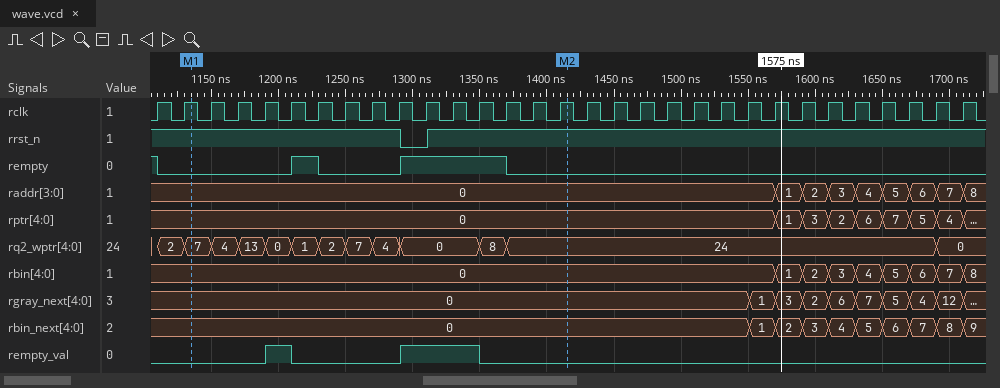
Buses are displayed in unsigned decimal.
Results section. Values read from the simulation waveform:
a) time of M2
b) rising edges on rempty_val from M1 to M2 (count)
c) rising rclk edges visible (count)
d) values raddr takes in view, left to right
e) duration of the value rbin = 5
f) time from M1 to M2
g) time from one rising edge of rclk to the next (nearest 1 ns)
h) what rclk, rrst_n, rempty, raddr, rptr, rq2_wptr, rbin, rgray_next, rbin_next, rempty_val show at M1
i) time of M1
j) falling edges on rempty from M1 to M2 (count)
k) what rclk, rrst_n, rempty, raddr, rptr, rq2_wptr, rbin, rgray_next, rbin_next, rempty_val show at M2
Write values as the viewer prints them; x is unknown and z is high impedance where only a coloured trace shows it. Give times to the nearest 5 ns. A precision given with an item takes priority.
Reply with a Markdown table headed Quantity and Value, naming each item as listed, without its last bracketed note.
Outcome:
| Quantity | Value |
|---|---|
| time of M2 | 1415 ns |
| rising edges on rempty_val from M1 to M2 | 2 |
| rising rclk edges visible | 31 |
| values raddr takes in view, left to right | 0, 1, 2, 3, 4, 5, 6, 7, 8 |
| duration of the value rbin = 5 | 20 ns |
| time from M1 to M2 | 280 ns |
| time from one rising edge of rclk to the next | 20 ns |
| what rclk, rrst_n, rempty, raddr, rptr, rq2_wptr, rbin, rgray_next, rbin_next, rempty_val show at M1 | rclk=1, rrst_n=1, rempty=0, raddr=0, rptr=0, rq2_wptr=7, rbin=0, rgray_next=0, rbin_next=0, rempty_val=0 |
| time of M1 | 1135 ns |
| falling edges on rempty from M1 to M2 | 2 |
| what rclk, rrst_n, rempty, raddr, rptr, rq2_wptr, rbin, rgray_next, rbin_next, rempty_val show at M2 | rclk=1, rrst_n=1, rempty=0, raddr=0, rptr=0, rq2_wptr=24, rbin=0, rgray_next=0, rbin_next=0, rempty_val=0 |
